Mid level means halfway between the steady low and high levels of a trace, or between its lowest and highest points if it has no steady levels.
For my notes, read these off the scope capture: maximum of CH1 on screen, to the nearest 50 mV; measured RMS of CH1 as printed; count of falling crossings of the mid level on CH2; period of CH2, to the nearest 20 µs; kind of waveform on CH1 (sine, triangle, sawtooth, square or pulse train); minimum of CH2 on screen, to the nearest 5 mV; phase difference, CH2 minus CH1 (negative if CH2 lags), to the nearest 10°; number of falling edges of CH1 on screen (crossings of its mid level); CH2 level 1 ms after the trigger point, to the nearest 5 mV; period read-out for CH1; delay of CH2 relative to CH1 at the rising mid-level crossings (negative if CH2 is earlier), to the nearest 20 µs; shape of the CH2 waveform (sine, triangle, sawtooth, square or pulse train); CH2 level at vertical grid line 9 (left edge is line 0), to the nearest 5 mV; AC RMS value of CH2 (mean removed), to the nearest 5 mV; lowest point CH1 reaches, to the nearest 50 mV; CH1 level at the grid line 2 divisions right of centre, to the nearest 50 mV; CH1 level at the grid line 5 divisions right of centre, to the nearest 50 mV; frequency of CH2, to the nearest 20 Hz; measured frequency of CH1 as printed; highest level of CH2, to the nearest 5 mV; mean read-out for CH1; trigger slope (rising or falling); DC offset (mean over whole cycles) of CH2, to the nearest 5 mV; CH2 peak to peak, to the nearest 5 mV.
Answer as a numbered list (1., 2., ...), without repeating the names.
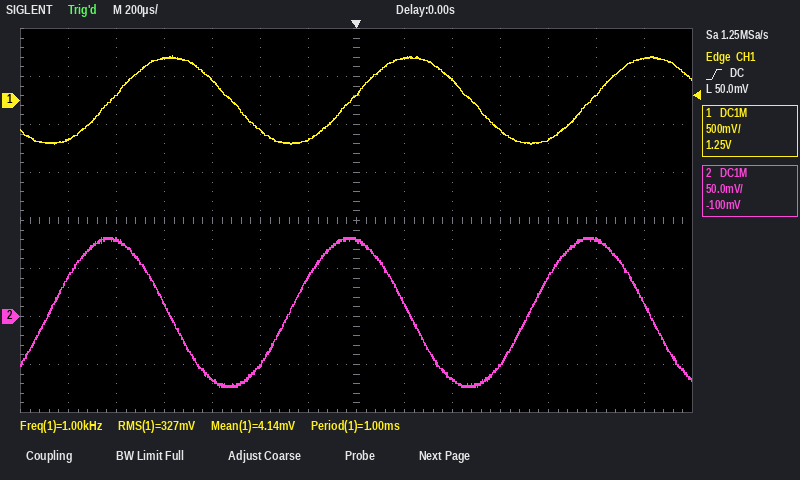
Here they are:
1. 450 mV
2. 327 mV
3. 3
4. 1.00 ms
5. sine
6. -75 mV
7. +90°
8. 2
9. 80 mV
10. 1.00 ms
11. -260 µs
12. sine
13. -65 mV
14. 55 mV
15. -450 mV
16. 200 mV
17. 50 mV
18. 1.00 kHz
19. 1.00 kHz
20. 80 mV
21. 4.14 mV
22. rising
23. 5 mV
24. 155 mV
